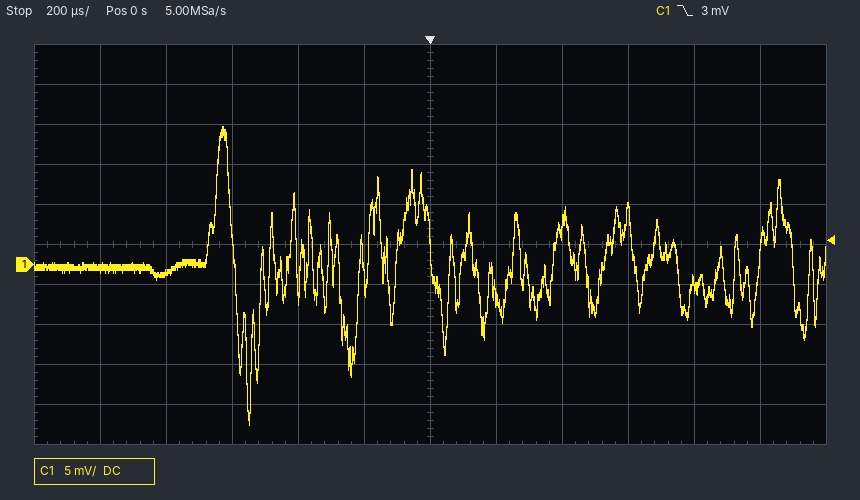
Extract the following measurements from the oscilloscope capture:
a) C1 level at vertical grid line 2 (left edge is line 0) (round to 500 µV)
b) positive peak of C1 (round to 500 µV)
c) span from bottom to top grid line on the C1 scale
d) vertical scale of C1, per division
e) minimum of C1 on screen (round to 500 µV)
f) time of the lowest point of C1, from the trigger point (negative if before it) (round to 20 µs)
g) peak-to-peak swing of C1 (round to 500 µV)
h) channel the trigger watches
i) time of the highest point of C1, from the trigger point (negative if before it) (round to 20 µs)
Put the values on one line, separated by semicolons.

-1.0 mV; 17.0 mV; 50 mV; 5 mV; -20.0 mV; -540 µs; 37.0 mV; C1; -620 µs
